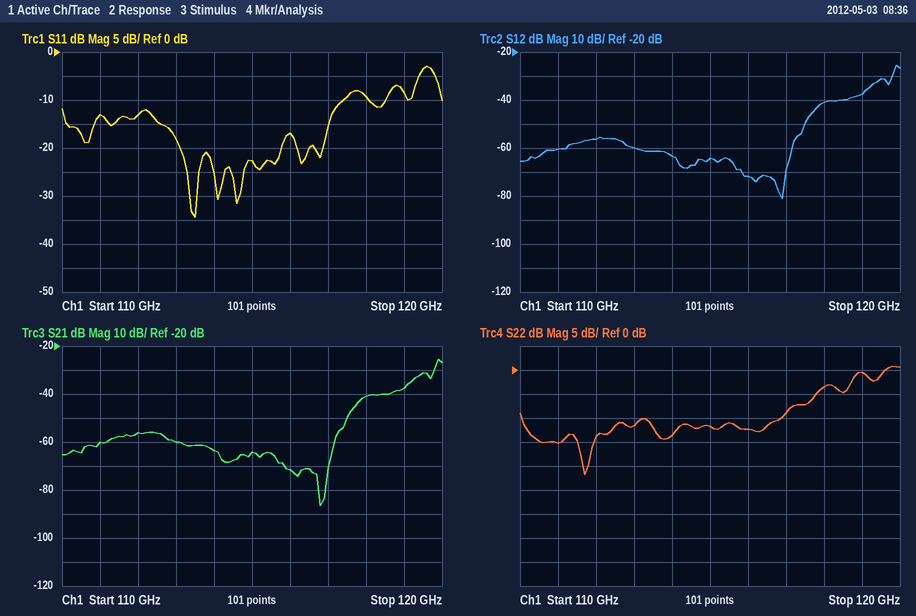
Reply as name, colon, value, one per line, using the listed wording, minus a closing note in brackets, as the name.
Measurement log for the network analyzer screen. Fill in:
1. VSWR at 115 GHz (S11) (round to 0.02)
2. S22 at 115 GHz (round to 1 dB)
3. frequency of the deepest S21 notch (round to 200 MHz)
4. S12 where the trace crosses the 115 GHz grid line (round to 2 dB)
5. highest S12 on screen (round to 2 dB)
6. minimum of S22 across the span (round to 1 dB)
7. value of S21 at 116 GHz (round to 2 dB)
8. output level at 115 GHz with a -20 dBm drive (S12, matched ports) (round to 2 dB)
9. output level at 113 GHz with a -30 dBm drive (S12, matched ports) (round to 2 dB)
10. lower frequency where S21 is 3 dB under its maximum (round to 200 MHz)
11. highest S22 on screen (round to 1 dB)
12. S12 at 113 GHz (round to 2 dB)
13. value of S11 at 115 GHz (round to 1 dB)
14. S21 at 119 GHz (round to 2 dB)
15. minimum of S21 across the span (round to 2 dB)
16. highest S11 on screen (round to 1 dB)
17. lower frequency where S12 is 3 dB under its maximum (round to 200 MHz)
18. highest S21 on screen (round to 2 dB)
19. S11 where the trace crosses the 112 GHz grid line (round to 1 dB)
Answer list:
VSWR at 115 GHz (S11): 1.16
S22 at 115 GHz: -12 dB
frequency of the deepest S21 notch: 116.8 GHz
S12 where the trace crosses the 115 GHz grid line: -64 dB
highest S12 on screen: -26 dB
minimum of S22 across the span: -22 dB
value of S21 at 116 GHz: -72 dB
output level at 115 GHz with a -20 dBm drive (S12, matched ports): -84 dBm
output level at 113 GHz with a -30 dBm drive (S12, matched ports): -90 dBm
lower frequency where S21 is 3 dB under its maximum: 119.8 GHz
highest S22 on screen: 1 dB
S12 at 113 GHz: -60 dB
value of S11 at 115 GHz: -23 dB
S21 at 119 GHz: -38 dB
minimum of S21 across the span: -86 dB
highest S11 on screen: -3 dB
lower frequency where S12 is 3 dB under its maximum: 119.8 GHz
highest S21 on screen: -26 dB
S11 where the trace crosses the 112 GHz grid line: -13 dB
